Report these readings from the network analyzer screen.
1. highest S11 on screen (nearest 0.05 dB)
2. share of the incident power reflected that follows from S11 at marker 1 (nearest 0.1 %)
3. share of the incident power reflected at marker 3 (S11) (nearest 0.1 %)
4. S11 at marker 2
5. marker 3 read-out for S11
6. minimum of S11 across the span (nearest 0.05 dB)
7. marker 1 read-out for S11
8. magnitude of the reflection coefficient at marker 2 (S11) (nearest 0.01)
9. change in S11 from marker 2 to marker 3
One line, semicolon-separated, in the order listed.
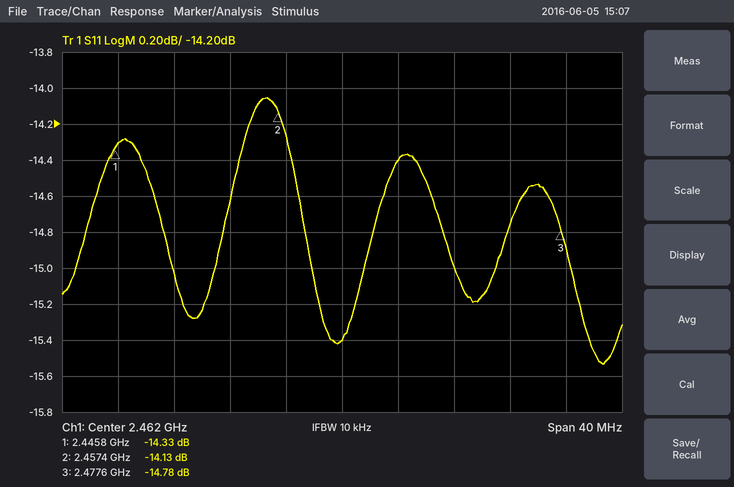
-14.05 dB; 3.7 %; 3.3 %; -14.13 dB; -14.78 dB; -15.55 dB; -14.33 dB; 0.20; -0.65 dB
